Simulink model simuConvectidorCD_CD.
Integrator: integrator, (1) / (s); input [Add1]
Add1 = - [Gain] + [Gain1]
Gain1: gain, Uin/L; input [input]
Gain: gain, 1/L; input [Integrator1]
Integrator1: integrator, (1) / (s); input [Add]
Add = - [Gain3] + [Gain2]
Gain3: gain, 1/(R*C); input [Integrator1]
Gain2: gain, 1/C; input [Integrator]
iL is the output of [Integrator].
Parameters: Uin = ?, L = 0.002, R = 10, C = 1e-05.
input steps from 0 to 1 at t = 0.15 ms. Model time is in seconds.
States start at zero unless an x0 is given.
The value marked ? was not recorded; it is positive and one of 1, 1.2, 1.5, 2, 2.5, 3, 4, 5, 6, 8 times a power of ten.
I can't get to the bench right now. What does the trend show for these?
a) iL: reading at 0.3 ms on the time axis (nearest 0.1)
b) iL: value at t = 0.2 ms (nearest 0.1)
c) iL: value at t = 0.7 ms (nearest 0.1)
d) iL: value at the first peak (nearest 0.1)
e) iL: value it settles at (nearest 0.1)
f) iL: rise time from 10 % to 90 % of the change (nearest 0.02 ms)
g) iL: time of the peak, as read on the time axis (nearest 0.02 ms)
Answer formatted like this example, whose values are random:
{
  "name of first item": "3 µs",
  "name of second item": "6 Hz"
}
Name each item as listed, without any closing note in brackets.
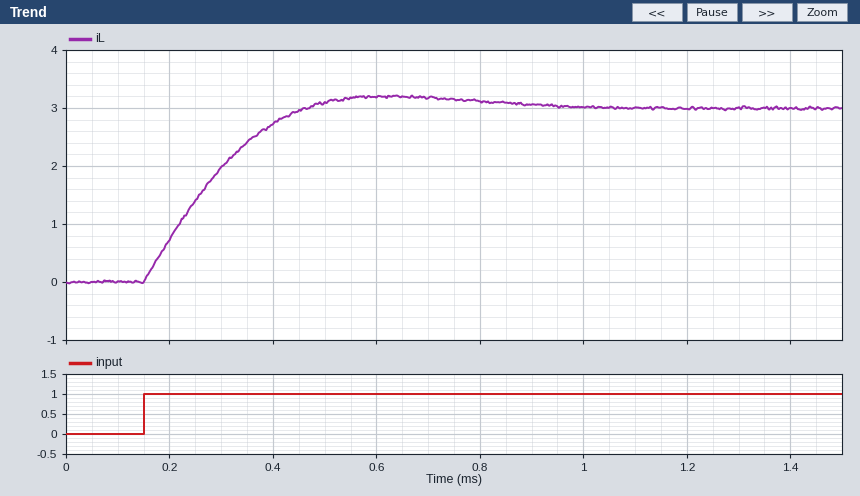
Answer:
{
  "iL: reading at 0.3 ms on the time axis": "2.0",
  "iL: value at t = 0.2 ms": "0.7",
  "iL: value at t = 0.7 ms": "3.2",
  "iL: value at the first peak": "3.2",
  "iL: value it settles at": "3.0",
  "iL: rise time from 10 % to 90 % of the change": "0.22 ms",
  "iL: time of the peak, as read on the time axis": "0.62 ms"
}
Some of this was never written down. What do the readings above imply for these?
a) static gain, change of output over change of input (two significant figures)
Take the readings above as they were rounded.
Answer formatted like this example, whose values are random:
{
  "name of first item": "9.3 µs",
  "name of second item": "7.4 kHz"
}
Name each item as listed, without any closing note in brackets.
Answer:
{
  "static gain, change of output over change of input": "3.0"
}
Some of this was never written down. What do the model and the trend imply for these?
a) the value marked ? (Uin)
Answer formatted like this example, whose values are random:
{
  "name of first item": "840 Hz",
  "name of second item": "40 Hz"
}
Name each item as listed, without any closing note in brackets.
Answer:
{
  "the value marked ?": "30"
}
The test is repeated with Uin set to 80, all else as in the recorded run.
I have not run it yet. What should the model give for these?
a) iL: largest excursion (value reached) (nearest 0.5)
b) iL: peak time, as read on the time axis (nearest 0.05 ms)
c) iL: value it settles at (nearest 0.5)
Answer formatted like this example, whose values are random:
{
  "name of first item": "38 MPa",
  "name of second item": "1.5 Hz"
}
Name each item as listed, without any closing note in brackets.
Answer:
{
  "iL: largest excursion (value reached)": "8.5",
  "iL: peak time, as read on the time axis": "0.60 ms",
  "iL: value it settles at": "8.0"
}
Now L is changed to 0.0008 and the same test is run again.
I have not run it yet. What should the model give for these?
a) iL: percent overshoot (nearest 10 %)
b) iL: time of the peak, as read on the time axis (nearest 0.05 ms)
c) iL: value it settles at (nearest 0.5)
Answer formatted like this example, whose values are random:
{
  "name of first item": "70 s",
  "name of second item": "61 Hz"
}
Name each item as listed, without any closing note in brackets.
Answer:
{
  "iL: percent overshoot": "40 %",
  "iL: time of the peak, as read on the time axis": "0.35 ms",
  "iL: value it settles at": "3.0"
}
